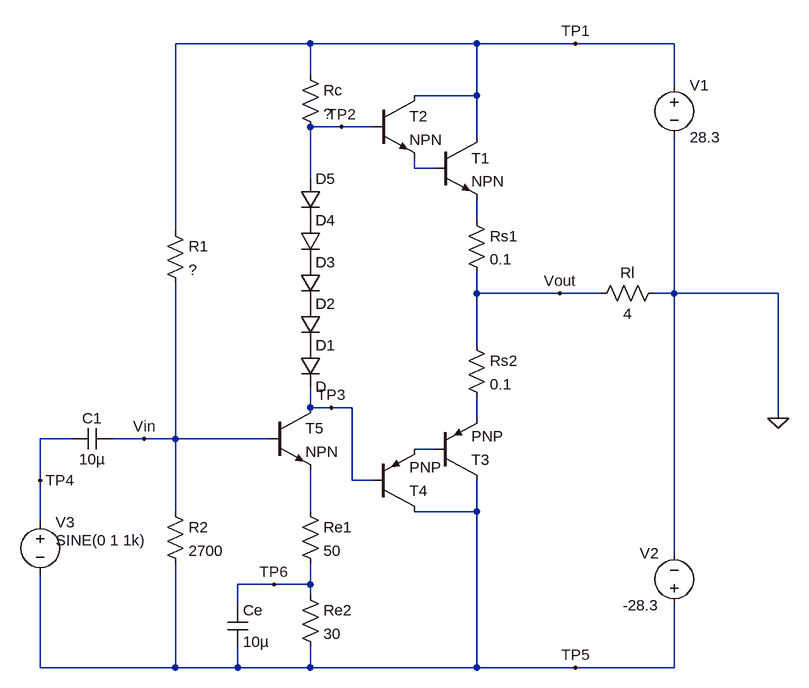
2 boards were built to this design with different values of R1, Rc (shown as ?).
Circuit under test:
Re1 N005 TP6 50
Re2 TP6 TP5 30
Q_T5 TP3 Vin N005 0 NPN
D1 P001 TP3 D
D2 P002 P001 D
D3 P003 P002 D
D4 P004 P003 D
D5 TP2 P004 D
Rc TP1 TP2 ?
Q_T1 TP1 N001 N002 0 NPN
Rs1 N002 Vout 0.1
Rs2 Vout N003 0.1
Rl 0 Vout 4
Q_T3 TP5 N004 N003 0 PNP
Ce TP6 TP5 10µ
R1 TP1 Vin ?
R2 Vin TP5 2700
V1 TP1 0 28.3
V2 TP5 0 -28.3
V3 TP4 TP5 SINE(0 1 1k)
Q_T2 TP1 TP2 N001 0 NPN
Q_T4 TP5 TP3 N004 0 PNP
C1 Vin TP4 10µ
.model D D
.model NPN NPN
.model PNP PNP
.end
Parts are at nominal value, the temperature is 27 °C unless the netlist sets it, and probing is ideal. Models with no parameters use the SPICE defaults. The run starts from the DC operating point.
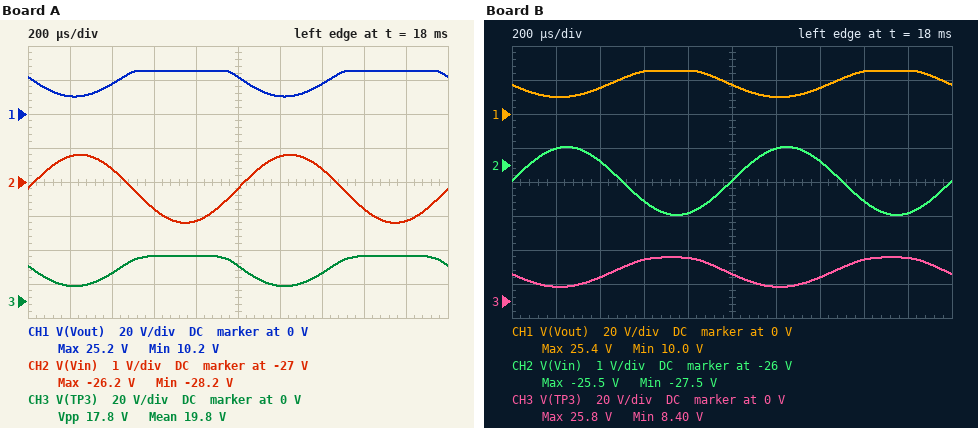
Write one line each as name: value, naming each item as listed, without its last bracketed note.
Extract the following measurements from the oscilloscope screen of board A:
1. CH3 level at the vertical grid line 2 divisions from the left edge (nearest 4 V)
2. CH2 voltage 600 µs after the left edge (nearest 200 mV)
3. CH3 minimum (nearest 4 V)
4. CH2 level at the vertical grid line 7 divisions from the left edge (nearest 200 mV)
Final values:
CH3 level at the vertical grid line 2 divisions from the left edge: 16 V
CH2 voltage 600 µs after the left edge: -27.8 V
CH3 minimum: 8 V
CH2 level at the vertical grid line 7 divisions from the left edge: -26.6 V
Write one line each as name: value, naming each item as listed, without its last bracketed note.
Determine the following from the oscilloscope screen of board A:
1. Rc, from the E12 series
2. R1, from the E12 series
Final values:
Rc, from the E12 series: 820 Ω
R1, from the E12 series: 120 kΩ
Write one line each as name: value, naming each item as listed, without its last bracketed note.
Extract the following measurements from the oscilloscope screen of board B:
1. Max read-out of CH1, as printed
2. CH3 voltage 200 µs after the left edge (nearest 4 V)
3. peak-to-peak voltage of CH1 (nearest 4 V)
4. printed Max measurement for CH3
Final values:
Max read-out of CH1, as printed: 25.4 V
CH3 voltage 200 µs after the left edge: 8 V
peak-to-peak voltage of CH1: 16 V
printed Max measurement for CH3: 25.8 V
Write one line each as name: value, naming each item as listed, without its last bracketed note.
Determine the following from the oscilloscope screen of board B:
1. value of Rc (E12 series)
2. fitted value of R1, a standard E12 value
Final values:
value of Rc: 560 Ω
fitted value of R1, a standard E12 value: 68 kΩ
